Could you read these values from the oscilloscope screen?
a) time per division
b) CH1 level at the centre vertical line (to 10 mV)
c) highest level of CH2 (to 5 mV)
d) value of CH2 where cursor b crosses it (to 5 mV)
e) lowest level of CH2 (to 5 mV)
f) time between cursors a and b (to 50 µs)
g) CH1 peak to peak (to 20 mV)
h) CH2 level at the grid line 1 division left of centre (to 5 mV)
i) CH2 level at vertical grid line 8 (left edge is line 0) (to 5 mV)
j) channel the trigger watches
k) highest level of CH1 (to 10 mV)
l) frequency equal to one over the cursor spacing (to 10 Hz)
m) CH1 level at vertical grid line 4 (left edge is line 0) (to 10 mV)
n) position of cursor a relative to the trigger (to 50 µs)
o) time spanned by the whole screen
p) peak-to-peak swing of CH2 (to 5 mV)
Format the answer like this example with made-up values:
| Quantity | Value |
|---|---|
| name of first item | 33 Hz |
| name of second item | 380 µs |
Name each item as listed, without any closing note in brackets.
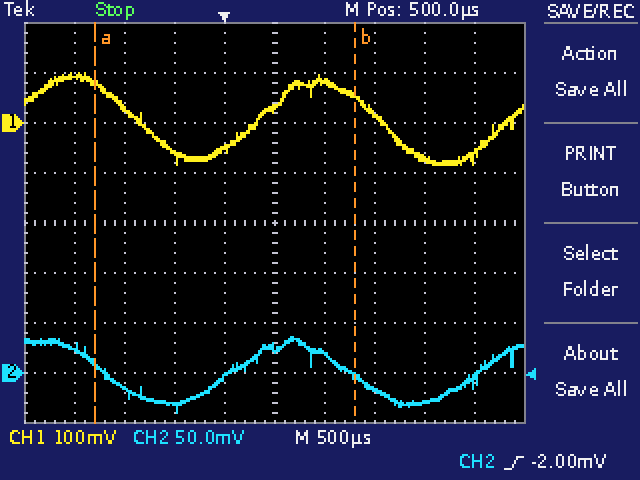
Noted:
| Quantity | Value |
|---|---|
| time per division | 500 µs |
| CH1 level at the centre vertical line | 30 mV |
| highest level of CH2 | 35 mV |
| value of CH2 where cursor b crosses it | -5 mV |
| lowest level of CH2 | -40 mV |
| time between cursors a and b | 2.60 ms |
| CH1 peak to peak | 180 mV |
| CH2 level at the grid line 1 division left of centre | -5 mV |
| CH2 level at vertical grid line 8 (left edge is line 0) | -30 mV |
| channel the trigger watches | CH2 |
| highest level of CH1 | 100 mV |
| frequency equal to one over the cursor spacing | 380 Hz |
| CH1 level at vertical grid line 4 (left edge is line 0) | -50 mV |
| position of cursor a relative to the trigger | -1.30 ms |
| time spanned by the whole screen | 5 ms |
| peak-to-peak swing of CH2 | 75 mV |
